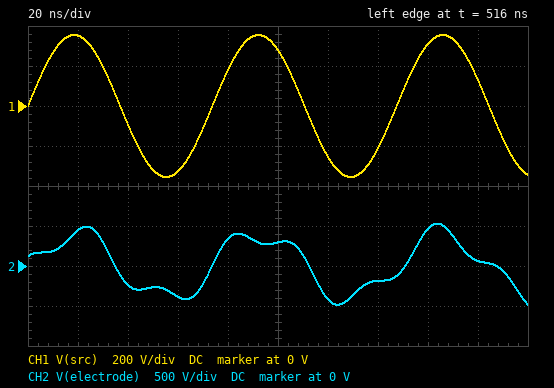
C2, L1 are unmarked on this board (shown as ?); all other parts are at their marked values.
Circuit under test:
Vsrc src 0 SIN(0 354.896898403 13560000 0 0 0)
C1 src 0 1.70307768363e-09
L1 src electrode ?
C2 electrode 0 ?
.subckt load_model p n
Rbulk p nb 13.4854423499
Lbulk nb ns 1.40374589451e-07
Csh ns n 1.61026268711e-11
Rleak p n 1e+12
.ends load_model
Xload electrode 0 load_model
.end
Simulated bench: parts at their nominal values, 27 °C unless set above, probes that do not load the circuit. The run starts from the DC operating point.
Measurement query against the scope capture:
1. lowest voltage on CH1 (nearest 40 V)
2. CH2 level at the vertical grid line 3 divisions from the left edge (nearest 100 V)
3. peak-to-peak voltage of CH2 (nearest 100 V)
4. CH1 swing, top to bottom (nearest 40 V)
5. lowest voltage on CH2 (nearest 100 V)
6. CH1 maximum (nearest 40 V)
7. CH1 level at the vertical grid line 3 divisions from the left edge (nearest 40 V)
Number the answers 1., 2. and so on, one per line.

1. -360 V
2. -400 V
3. 1.0 kV
4. 720 V
5. -500 V
6. 360 V
7. -320 V
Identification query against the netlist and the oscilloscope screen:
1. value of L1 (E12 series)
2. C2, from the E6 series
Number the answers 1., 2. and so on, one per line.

1. 39 nH
2. 470 pF
